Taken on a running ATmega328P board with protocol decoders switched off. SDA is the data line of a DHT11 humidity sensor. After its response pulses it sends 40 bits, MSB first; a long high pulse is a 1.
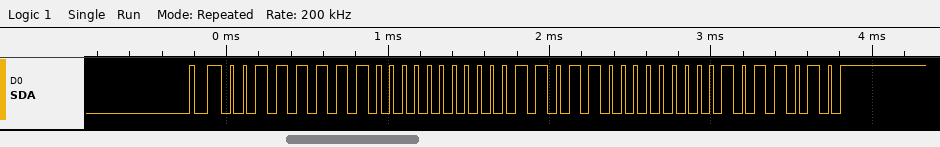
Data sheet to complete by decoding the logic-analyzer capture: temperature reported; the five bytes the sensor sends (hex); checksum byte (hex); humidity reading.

27.0 °C
3F 00 1B 00 5A
0x5A
63 %
